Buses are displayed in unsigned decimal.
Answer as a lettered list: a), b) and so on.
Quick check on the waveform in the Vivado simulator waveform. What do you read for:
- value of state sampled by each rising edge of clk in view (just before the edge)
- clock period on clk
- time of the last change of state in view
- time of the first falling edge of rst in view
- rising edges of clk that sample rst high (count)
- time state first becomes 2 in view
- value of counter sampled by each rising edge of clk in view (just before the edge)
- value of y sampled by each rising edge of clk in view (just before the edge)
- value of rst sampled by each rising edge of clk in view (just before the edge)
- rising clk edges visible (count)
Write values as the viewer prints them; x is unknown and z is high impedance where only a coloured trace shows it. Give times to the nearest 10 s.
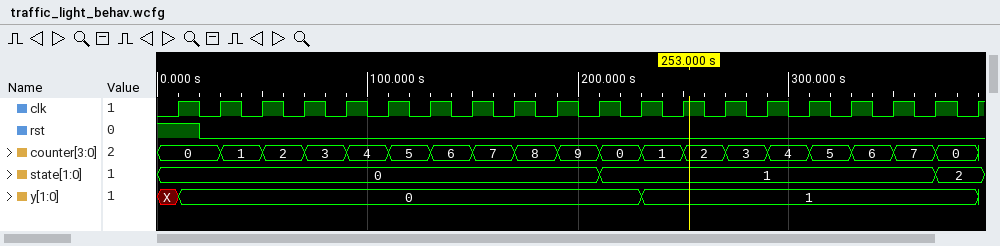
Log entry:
a) 0, 0, 0, 0, 0, 0, 0, 0, 0, 0, 0, 1, 1, 1, 1, 1, 1, 1, 1, 2
b) 20 s
c) 370 s
d) 20 s
e) 1
f) 370 s
g) 0, 0, 1, 2, 3, 4, 5, 6, 7, 8, 9, 0, 1, 2, 3, 4, 5, 6, 7, 0
h) X, 0, 0, 0, 0, 0, 0, 0, 0, 0, 0, 0, 1, 1, 1, 1, 1, 1, 1, 1
i) 1 0 0 0 0 0 0 0 0 0 0 0 0 0 0 0 0 0 0 0
j) 20
